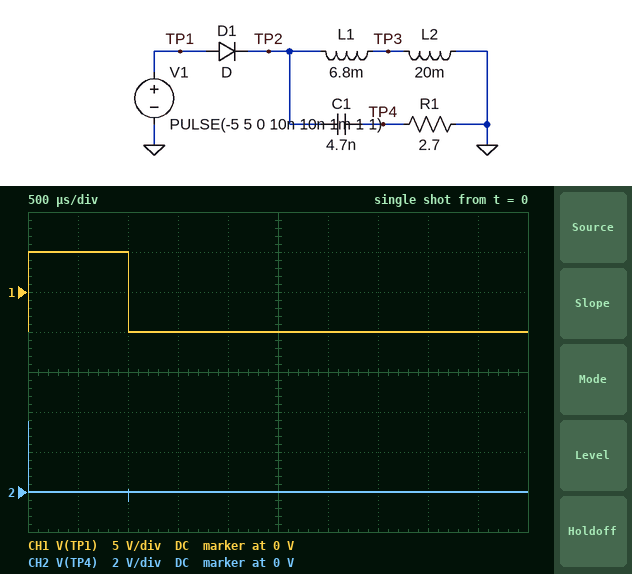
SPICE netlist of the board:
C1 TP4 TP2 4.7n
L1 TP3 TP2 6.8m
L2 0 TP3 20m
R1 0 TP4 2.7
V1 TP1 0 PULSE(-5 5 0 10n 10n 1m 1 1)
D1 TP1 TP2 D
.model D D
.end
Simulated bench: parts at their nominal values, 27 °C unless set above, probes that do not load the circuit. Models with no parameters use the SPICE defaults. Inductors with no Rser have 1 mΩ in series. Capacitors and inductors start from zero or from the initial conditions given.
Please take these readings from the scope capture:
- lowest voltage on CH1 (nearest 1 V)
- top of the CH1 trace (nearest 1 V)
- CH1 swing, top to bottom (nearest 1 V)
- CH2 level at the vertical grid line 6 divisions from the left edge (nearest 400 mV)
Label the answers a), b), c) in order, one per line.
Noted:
a) -5 V
b) 5 V
c) 10 V
d) 0 V
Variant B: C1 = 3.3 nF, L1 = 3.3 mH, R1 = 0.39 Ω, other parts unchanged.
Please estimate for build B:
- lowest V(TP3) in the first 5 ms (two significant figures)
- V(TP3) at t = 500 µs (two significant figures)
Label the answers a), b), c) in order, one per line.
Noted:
a) -5.0 V
b) 3.6 V
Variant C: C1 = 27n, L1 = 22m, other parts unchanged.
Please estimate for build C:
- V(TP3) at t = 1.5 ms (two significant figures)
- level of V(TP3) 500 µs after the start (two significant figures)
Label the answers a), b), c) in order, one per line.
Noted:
a) -2.7 V
b) 2.0 V
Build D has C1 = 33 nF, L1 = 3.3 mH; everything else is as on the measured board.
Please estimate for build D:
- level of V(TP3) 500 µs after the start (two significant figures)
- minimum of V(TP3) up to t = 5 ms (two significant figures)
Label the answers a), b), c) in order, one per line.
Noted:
a) 3.6 V
b) -5.0 V
